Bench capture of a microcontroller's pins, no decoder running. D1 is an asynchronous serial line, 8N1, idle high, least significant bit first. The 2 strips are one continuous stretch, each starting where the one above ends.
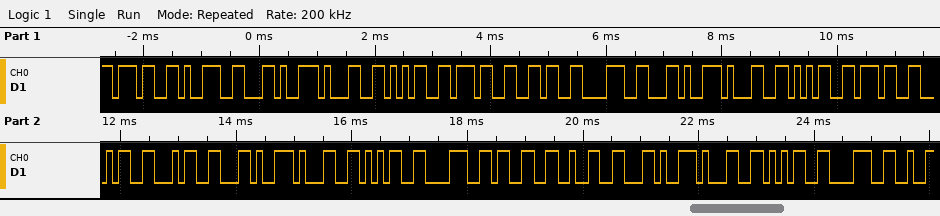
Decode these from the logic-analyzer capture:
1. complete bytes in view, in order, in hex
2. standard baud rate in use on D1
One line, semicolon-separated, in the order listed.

37 39 2C 31 35 37 36 38 2C 31 35 37 34 34 2C 31 35 38 33 32 2C 31 35 38; 9600 baud
